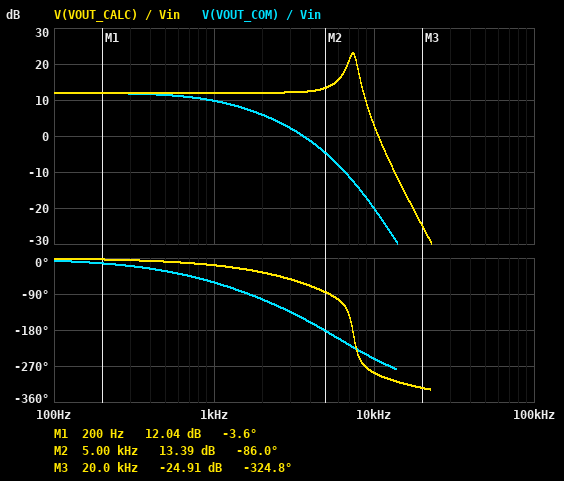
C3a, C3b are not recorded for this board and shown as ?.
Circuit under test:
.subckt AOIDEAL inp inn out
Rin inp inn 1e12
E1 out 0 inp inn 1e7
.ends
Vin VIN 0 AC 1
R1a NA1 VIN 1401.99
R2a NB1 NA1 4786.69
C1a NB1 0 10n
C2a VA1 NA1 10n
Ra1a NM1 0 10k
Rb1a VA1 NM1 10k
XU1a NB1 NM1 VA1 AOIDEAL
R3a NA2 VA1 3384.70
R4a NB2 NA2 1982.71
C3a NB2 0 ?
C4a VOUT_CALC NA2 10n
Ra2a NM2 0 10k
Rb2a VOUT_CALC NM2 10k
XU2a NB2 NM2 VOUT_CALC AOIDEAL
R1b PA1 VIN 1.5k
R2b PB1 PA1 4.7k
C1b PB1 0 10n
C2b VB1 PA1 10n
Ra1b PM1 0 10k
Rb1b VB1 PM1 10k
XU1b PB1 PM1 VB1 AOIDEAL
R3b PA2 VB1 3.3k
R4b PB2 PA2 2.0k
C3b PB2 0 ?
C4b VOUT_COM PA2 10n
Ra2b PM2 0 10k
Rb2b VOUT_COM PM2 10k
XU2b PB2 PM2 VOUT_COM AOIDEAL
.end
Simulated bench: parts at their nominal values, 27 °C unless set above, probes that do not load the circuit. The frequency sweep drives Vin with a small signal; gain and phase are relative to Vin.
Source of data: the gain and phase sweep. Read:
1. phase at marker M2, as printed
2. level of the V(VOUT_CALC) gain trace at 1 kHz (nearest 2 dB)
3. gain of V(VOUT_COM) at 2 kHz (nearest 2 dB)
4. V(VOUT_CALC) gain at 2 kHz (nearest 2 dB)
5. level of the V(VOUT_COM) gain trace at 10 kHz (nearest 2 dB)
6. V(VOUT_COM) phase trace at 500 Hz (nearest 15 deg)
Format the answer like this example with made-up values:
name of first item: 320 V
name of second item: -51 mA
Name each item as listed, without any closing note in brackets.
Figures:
phase at marker M2, as printed: -86.0 deg
level of the V(VOUT_CALC) gain trace at 1 kHz: 12 dB
gain of V(VOUT_COM) at 2 kHz: 6 dB
V(VOUT_CALC) gain at 2 kHz: 12 dB
level of the V(VOUT_COM) gain trace at 10 kHz: -20 dB
V(VOUT_COM) phase trace at 500 Hz: -30 deg
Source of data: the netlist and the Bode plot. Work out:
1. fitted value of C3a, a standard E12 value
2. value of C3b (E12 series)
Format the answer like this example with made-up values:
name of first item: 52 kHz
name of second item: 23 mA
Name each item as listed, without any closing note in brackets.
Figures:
fitted value of C3a, a standard E12 value: 6.8 nF
value of C3b: 33 nF
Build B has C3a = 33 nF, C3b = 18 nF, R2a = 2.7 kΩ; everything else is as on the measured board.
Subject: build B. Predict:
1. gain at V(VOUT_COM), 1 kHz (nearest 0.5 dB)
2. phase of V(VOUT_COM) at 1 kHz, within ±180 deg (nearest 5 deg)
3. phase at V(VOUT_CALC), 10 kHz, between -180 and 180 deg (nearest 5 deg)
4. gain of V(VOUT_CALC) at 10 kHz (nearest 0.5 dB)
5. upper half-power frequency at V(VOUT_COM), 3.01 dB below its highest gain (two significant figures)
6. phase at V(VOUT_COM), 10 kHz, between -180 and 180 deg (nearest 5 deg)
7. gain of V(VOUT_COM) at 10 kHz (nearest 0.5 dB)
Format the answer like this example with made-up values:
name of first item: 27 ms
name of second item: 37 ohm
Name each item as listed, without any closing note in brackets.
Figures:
gain at V(VOUT_COM), 1 kHz: 11.5 dB
phase of V(VOUT_COM) at 1 kHz, within ±180 deg: -40 deg
phase at V(VOUT_CALC), 10 kHz, between -180 and 180 deg: 125 deg
gain of V(VOUT_CALC) at 10 kHz: -14.5 dB
upper half-power frequency at V(VOUT_COM), 3.01 dB below its highest gain: 2.7 kHz
phase at V(VOUT_COM), 10 kHz, between -180 and 180 deg: 105 deg
gain of V(VOUT_COM) at 10 kHz: -13.5 dB
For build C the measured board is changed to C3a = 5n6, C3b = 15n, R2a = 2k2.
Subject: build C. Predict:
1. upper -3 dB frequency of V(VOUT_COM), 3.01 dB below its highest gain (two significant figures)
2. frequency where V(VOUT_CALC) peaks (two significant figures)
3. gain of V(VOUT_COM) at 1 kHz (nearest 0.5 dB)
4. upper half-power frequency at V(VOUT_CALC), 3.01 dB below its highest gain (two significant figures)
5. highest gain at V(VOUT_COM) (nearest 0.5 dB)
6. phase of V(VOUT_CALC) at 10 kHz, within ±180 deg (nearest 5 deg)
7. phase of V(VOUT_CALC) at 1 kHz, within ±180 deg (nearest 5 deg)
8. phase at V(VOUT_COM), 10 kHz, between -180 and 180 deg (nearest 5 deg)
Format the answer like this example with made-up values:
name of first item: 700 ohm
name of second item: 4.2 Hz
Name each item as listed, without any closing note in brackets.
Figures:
upper -3 dB frequency of V(VOUT_COM), 3.01 dB below its highest gain: 3.5 kHz
frequency where V(VOUT_CALC) peaks: 8.1 kHz
gain of V(VOUT_COM) at 1 kHz: 12.0 dB
upper half-power frequency at V(VOUT_CALC), 3.01 dB below its highest gain: 8.8 kHz
highest gain at V(VOUT_COM): 12.0 dB
phase of V(VOUT_CALC) at 10 kHz, within ±180 deg: 55 deg
phase of V(VOUT_CALC) at 1 kHz, within ±180 deg: -5 deg
phase at V(VOUT_COM), 10 kHz, between -180 and 180 deg: 105 deg
